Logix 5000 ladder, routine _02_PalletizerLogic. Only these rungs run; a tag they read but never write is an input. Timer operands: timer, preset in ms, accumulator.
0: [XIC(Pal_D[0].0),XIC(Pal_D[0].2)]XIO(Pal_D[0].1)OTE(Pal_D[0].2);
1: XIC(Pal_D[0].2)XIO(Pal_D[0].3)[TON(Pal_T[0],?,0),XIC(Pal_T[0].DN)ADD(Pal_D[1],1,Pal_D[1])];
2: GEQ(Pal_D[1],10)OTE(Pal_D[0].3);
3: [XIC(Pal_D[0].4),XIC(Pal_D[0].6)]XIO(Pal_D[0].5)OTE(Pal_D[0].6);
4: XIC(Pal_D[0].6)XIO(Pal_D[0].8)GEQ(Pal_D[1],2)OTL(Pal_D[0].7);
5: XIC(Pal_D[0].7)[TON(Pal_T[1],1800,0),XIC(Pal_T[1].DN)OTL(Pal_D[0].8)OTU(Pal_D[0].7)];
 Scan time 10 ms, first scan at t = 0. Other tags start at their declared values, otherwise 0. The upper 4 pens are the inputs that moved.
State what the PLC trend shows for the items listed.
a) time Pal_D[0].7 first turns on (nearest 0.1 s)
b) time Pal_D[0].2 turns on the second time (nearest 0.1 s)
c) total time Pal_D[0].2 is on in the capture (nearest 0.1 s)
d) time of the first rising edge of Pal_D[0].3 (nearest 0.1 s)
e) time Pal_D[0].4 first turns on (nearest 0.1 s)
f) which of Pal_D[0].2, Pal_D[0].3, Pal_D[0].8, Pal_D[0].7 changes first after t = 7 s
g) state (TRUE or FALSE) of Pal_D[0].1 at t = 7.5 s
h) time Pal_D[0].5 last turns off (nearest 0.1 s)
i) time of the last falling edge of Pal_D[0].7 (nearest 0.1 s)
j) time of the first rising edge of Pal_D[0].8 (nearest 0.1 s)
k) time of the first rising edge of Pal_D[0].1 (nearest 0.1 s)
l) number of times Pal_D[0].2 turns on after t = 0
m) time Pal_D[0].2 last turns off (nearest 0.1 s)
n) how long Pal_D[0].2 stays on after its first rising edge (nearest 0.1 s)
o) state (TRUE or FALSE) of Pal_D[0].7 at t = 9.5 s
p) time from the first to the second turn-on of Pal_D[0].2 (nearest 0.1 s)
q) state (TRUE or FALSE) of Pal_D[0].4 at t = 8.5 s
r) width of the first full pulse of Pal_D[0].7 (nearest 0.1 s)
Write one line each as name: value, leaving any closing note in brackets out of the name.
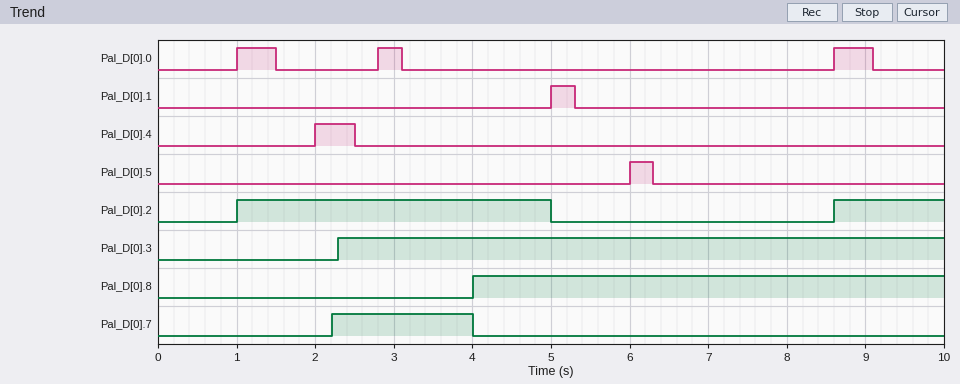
time Pal_D[0].7 first turns on: 2.2 s
time Pal_D[0].2 turns on the second time: 8.6 s
total time Pal_D[0].2 is on in the capture: 5.4 s
time of the first rising edge of Pal_D[0].3: 2.3 s
time Pal_D[0].4 first turns on: 2.0 s
which of Pal_D[0].2, Pal_D[0].3, Pal_D[0].8, Pal_D[0].7 changes first after t = 7 s: Pal_D[0].2
state (TRUE or FALSE) of Pal_D[0].1 at t = 7.5 s: FALSE
time Pal_D[0].5 last turns off: 6.3 s
time of the last falling edge of Pal_D[0].7: 4.0 s
time of the first rising edge of Pal_D[0].8: 4.0 s
time of the first rising edge of Pal_D[0].1: 5.0 s
number of times Pal_D[0].2 turns on after t = 0: 2
time Pal_D[0].2 last turns off: 5.0 s
how long Pal_D[0].2 stays on after its first rising edge: 4.0 s
state (TRUE or FALSE) of Pal_D[0].7 at t = 9.5 s: FALSE
time from the first to the second turn-on of Pal_D[0].2: 7.6 s
state (TRUE or FALSE) of Pal_D[0].4 at t = 8.5 s: FALSE
width of the first full pulse of Pal_D[0].7: 1.8 s
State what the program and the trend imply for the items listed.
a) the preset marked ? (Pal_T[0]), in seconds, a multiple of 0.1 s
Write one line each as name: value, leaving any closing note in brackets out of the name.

the preset marked ? (Pal_T[0]), in seconds, a multiple of 0.1 s: 1.2 s
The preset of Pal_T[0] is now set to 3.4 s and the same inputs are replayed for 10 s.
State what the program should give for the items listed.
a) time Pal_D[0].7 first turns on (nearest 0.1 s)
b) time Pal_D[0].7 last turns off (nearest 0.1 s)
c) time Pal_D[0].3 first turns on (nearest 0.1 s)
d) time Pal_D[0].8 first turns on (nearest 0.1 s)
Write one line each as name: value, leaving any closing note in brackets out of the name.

time Pal_D[0].7 first turns on: 4.4 s
time Pal_D[0].7 last turns off: 6.2 s
time Pal_D[0].3 first turns on: 4.5 s
time Pal_D[0].8 first turns on: 6.2 s
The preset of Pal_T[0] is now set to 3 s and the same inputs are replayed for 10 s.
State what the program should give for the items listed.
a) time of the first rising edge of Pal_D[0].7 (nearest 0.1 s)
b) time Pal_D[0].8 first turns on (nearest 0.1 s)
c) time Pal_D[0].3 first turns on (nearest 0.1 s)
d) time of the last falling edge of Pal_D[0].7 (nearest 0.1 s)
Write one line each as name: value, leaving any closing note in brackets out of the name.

time of the first rising edge of Pal_D[0].7: 4.0 s
time Pal_D[0].8 first turns on: 5.8 s
time Pal_D[0].3 first turns on: 4.1 s
time of the last falling edge of Pal_D[0].7: 5.8 s
